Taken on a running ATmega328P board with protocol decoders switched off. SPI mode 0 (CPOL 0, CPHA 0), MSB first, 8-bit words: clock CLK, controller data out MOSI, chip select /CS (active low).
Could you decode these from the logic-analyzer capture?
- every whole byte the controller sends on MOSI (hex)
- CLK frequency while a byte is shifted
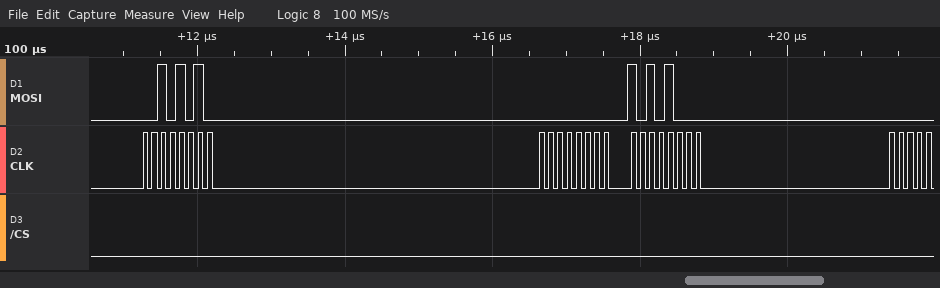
2A 00 A8
8 MHz
